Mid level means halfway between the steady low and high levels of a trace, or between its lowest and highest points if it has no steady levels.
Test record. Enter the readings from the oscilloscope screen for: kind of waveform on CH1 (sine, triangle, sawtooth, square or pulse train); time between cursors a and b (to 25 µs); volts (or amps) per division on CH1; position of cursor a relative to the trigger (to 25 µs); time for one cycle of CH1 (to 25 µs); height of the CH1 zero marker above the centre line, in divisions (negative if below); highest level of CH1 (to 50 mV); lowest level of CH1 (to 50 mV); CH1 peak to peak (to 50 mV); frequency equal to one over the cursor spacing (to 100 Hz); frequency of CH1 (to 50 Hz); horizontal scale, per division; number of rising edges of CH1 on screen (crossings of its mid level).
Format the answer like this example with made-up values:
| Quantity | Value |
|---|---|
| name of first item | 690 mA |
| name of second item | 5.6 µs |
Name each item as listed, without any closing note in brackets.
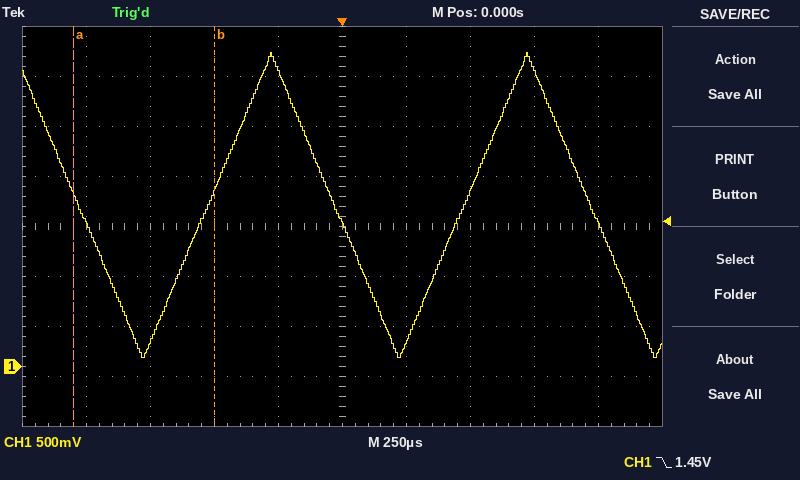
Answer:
| Quantity | Value |
|---|---|
| kind of waveform on CH1 | triangle |
| time between cursors a and b | 550 µs |
| volts (or amps) per division on CH1 | 500 mV |
| position of cursor a relative to the trigger | -1.050 ms |
| time for one cycle of CH1 | 1.000 ms |
| height of the CH1 zero marker above the centre line, in divisions | -2.8 div |
| highest level of CH1 | 3.15 V |
| lowest level of CH1 | 100 mV |
| CH1 peak to peak | 3.05 V |
| frequency equal to one over the cursor spacing | 1.8 kHz |
| frequency of CH1 | 1.00 kHz |
| horizontal scale, per division | 250 µs |
| number of rising edges of CH1 on screen | 2 |
